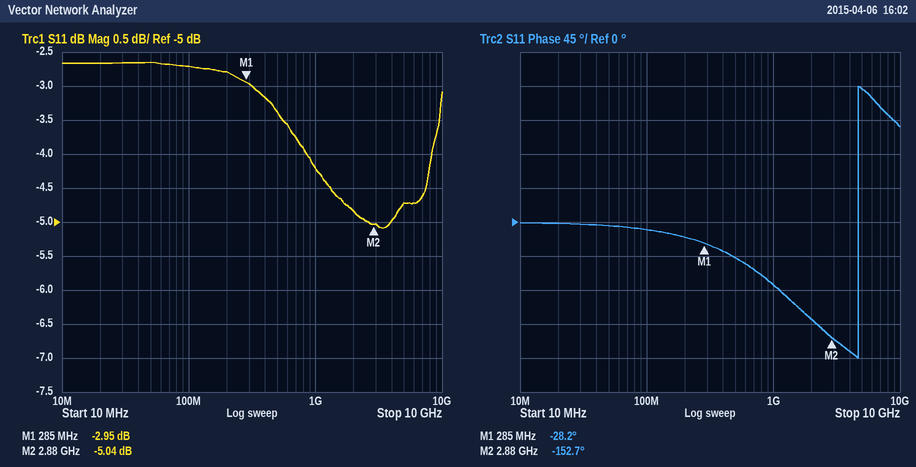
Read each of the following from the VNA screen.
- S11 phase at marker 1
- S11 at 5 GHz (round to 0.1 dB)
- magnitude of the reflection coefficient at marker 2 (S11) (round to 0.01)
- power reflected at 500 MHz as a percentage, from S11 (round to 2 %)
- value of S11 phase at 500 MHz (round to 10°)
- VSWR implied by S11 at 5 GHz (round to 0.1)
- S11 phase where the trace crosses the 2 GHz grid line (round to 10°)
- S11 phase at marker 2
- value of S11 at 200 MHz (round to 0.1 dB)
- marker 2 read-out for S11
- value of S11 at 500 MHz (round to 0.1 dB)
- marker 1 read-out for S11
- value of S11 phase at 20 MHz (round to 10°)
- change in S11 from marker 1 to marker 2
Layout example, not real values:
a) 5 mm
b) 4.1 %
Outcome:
a) -28.2°
b) -4.7 dB
c) 0.56
d) 46 %
e) -50°
f) 3.8
g) -130°
h) -152.7°
i) -2.8 dB
j) -5.04 dB
k) -3.4 dB
l) -2.95 dB
m) 0°
n) -2.09 dB
